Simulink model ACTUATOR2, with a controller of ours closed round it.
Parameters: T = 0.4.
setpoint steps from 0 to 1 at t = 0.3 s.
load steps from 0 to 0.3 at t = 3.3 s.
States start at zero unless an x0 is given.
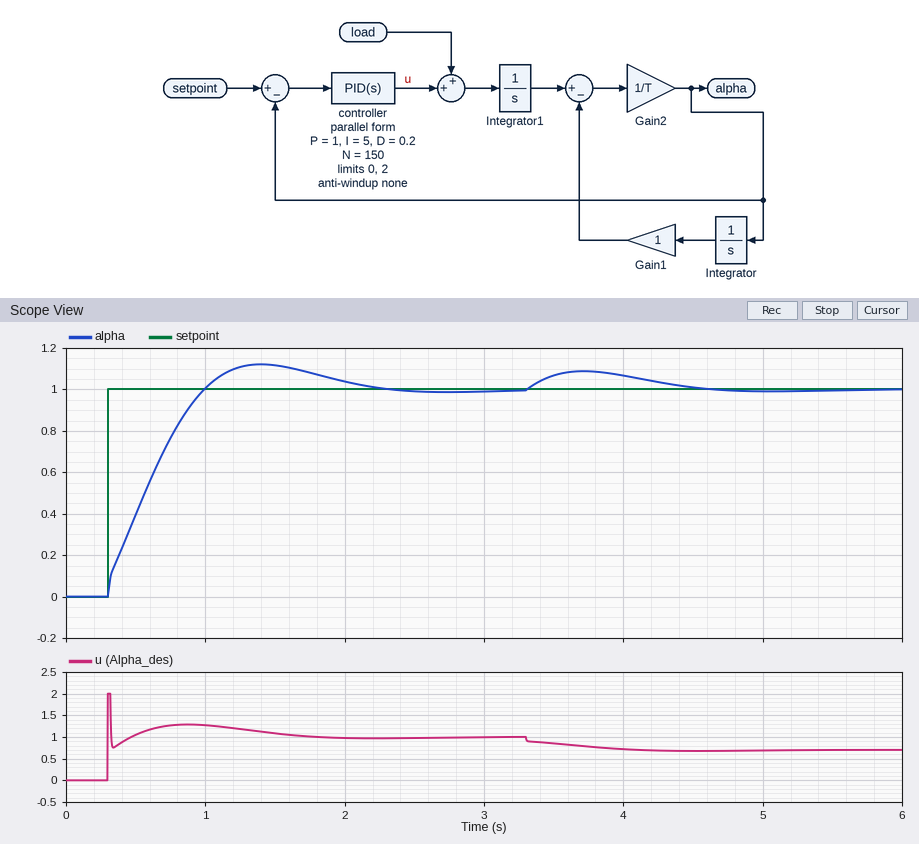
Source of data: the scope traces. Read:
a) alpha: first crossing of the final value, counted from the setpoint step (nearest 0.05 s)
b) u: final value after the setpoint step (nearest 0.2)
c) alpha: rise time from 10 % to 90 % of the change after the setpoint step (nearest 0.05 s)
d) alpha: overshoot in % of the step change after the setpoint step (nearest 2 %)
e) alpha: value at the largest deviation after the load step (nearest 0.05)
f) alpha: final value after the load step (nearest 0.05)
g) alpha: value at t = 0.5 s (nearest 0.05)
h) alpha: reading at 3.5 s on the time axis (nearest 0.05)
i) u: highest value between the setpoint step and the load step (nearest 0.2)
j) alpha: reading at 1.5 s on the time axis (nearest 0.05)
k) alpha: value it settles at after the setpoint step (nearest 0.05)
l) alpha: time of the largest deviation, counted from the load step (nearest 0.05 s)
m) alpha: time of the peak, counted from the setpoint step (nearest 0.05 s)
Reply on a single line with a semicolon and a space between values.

0.70 s; 1.0; 0.55 s; 12 %; 1.10; 1.00; 0.40; 1.05; 2.0; 1.10; 1.00; 0.40 s; 1.10 s
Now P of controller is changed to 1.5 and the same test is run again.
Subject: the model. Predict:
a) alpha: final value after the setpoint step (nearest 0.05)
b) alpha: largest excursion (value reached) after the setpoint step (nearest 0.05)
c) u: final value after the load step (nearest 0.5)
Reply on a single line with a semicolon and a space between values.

1.00; 1.05; 0.5
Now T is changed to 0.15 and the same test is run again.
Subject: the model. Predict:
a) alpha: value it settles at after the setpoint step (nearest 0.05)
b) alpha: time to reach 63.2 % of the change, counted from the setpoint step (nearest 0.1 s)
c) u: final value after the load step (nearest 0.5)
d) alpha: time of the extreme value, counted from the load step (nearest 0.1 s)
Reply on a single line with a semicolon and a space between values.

1.00; 0.3 s; 0.5; 0.3 s
